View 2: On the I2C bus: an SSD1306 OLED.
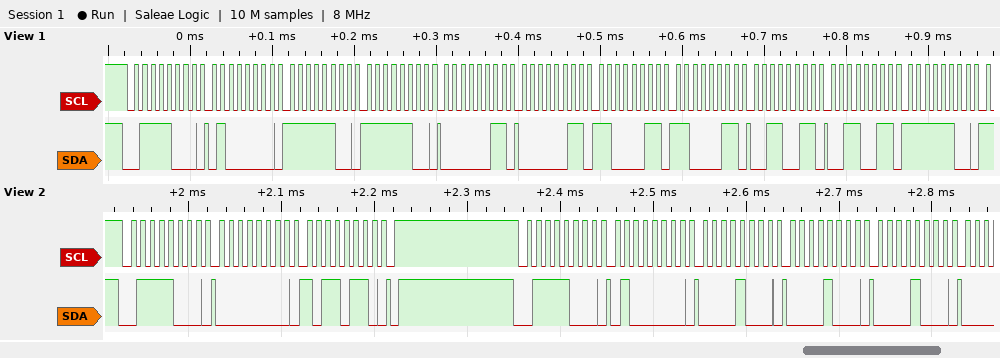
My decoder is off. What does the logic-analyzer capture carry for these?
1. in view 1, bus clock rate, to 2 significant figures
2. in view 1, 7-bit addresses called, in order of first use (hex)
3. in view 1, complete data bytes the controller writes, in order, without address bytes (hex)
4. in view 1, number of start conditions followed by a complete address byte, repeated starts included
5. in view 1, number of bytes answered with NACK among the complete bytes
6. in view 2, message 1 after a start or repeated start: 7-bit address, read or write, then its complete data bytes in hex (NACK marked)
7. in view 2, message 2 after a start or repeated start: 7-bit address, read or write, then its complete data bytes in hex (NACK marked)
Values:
100 kHz
0x3C
40 FC FC 03 03 C3 C3 33 33 FC
1
0
0x3C write: 00 B6
0x3C write: 40 08 08 08
